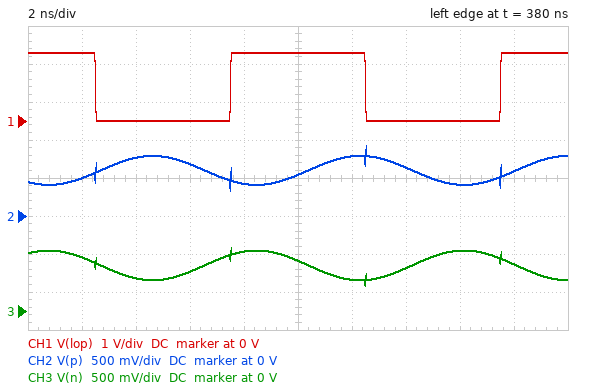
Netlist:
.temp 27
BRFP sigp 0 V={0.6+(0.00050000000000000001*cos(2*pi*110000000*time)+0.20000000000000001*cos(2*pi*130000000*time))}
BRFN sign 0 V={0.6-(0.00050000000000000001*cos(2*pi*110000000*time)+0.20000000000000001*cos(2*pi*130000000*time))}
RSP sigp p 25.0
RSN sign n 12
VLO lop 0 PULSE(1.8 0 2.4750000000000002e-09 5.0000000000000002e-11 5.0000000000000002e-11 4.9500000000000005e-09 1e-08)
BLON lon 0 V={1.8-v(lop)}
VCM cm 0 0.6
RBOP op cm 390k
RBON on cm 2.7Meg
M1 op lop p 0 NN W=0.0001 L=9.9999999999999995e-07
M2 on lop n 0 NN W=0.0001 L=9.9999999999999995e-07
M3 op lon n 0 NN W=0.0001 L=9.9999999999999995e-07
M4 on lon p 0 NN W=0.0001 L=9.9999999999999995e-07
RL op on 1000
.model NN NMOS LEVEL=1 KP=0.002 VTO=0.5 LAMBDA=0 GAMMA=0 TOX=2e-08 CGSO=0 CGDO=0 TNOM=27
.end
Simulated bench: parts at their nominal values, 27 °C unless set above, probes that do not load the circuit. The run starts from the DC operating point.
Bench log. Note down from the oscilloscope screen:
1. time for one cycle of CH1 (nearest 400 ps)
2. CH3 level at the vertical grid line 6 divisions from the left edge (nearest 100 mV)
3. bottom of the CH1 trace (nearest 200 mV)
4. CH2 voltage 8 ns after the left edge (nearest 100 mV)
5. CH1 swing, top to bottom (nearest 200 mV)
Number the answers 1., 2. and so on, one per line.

1. 10.0 ns
2. 400 mV
3. 0 V
4. 400 mV
5. 1.8 V
